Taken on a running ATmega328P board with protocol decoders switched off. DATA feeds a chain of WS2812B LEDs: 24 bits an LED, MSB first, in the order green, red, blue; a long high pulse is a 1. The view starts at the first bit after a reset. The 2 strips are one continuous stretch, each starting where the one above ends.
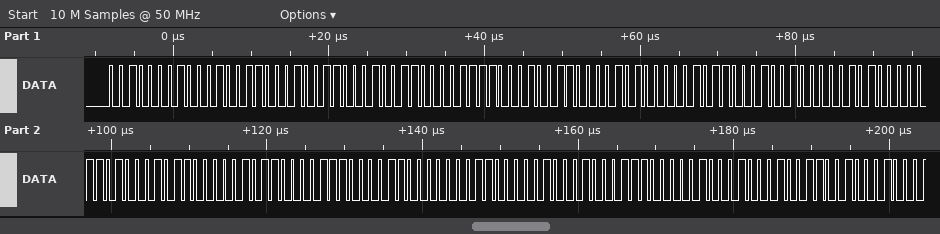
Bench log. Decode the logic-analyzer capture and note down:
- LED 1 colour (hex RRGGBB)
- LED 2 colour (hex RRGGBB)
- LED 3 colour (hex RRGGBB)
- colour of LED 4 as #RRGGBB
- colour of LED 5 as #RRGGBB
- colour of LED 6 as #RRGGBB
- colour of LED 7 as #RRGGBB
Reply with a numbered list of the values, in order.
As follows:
1. #132113
2. #0F1313
3. #0B0A12
4. #0D0A16
5. #0E0B18
6. #110C1C
7. #131122
